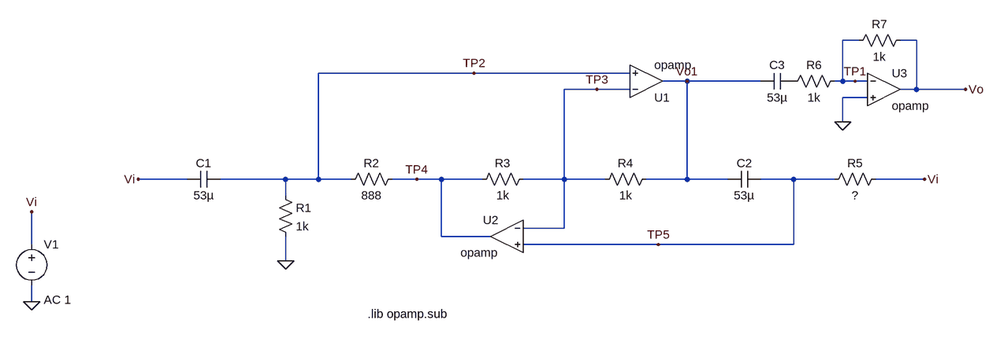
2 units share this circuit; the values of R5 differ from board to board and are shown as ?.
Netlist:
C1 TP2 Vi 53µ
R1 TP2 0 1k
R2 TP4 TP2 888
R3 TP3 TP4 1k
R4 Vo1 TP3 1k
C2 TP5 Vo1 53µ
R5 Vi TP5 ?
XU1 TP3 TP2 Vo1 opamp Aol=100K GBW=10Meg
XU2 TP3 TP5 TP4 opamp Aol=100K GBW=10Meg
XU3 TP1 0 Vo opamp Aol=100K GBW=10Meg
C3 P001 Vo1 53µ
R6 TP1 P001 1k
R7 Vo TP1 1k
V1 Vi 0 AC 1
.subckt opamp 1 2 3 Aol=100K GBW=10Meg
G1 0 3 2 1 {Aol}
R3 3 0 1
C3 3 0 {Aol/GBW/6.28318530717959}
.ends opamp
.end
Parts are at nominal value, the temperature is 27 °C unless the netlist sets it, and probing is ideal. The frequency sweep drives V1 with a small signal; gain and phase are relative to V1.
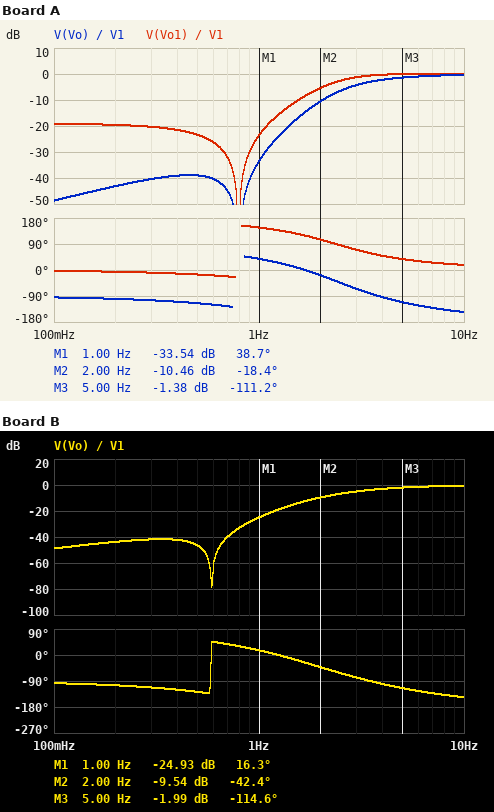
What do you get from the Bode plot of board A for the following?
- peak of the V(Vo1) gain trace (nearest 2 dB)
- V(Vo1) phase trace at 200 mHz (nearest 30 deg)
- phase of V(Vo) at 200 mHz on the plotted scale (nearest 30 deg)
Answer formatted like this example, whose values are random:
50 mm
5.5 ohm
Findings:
0 dB
0 deg
-90 deg
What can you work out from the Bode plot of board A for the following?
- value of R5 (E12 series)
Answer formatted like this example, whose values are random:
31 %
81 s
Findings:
1.8 kΩ
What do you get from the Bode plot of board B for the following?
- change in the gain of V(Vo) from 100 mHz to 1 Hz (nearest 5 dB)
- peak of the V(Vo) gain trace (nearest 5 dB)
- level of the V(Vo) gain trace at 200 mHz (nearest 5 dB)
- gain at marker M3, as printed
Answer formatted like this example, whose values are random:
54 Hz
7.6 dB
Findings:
25 dB
0 dB
-45 dB
-1.99 dB
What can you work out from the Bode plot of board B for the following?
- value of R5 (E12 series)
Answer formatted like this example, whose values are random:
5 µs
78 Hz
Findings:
3.3 kΩ
